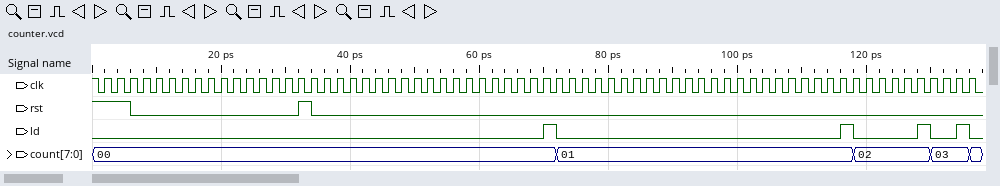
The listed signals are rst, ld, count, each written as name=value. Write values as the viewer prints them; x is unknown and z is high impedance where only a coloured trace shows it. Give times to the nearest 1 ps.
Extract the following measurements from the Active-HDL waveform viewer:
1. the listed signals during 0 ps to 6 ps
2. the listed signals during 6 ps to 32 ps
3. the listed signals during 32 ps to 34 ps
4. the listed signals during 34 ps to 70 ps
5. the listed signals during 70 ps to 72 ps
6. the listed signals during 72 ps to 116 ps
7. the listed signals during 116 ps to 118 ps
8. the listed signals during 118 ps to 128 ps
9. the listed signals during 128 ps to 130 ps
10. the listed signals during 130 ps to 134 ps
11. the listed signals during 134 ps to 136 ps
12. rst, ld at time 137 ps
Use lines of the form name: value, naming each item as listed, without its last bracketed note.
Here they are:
the listed signals during 0 ps to 6 ps: rst=1, ld=0, count=00
the listed signals during 6 ps to 32 ps: rst=0, ld=0, count=00
the listed signals during 32 ps to 34 ps: rst=1, ld=0, count=00
the listed signals during 34 ps to 70 ps: rst=0, ld=0, count=00
the listed signals during 70 ps to 72 ps: rst=0, ld=1, count=00
the listed signals during 72 ps to 116 ps: rst=0, ld=0, count=01
the listed signals during 116 ps to 118 ps: rst=0, ld=1, count=01
the listed signals during 118 ps to 128 ps: rst=0, ld=0, count=02
the listed signals during 128 ps to 130 ps: rst=0, ld=1, count=02
the listed signals during 130 ps to 134 ps: rst=0, ld=0, count=03
the listed signals during 134 ps to 136 ps: rst=0, ld=1, count=03
rst, ld at time 137 ps: rst=0, ld=0
